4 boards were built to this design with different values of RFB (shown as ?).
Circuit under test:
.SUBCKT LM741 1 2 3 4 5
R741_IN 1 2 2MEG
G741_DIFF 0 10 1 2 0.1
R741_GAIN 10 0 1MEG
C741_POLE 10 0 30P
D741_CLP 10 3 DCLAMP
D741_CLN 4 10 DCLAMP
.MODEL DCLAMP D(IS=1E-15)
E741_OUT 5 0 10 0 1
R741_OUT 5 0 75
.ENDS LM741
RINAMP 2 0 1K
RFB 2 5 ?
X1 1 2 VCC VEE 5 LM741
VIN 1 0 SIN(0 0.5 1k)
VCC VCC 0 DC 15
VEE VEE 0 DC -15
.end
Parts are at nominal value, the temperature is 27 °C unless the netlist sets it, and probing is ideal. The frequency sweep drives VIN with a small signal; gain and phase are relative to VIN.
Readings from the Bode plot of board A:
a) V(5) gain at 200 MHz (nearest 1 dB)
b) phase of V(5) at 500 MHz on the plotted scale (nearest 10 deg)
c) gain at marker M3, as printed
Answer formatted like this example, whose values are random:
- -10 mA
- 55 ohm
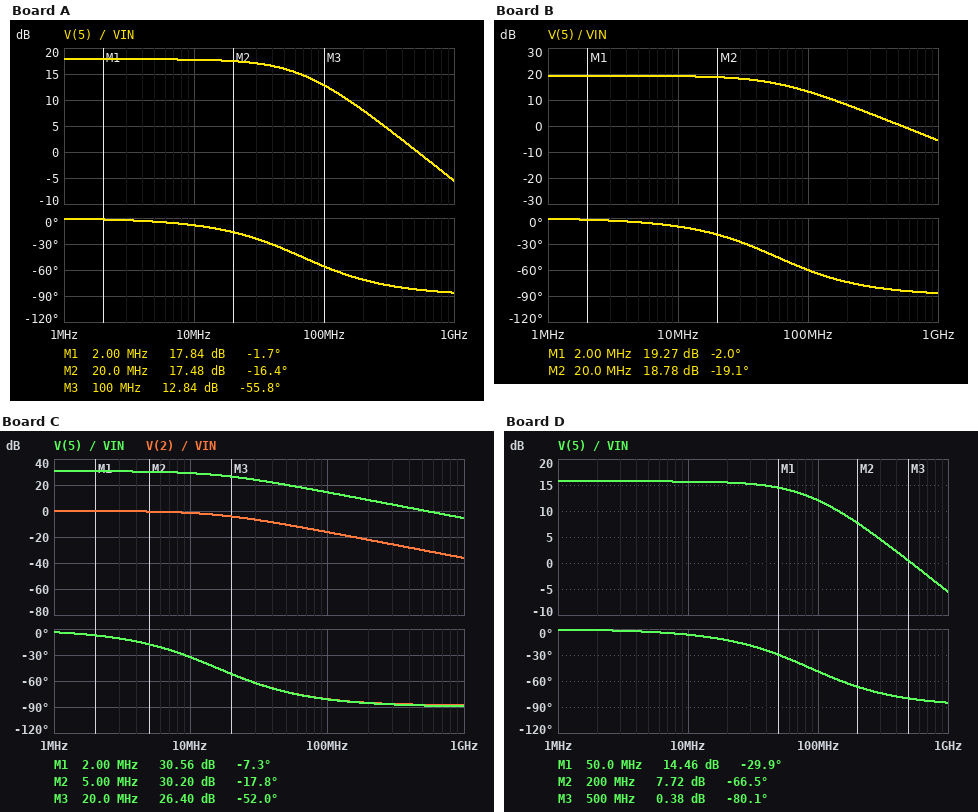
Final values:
- 8 dB
- -80 deg
- 12.84 dB
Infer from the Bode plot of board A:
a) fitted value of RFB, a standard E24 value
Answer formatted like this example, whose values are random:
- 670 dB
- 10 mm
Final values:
- 6.8 kΩ
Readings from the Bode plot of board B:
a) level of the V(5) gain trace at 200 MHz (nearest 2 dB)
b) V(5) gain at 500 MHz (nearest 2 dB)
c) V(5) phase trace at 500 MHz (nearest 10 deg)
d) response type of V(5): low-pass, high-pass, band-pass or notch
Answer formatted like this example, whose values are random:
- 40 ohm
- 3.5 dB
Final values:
- 8 dB
- 0 dB
- -80 deg
- low-pass
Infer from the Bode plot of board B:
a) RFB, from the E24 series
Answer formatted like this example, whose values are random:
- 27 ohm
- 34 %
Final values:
- 8.2 kΩ
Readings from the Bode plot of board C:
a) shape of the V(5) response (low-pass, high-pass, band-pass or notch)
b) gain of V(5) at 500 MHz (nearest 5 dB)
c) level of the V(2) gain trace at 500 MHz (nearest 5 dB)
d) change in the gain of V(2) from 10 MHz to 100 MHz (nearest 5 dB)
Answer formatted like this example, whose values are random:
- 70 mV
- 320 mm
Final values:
- low-pass
- 0 dB
- -30 dB
- -15 dB
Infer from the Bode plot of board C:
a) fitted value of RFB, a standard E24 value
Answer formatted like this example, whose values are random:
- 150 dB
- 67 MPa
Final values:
- 33 kΩ
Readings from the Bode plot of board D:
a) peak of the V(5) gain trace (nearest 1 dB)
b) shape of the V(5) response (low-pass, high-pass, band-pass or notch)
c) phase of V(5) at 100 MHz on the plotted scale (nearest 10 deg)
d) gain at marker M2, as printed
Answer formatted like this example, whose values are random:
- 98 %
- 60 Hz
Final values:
- 16 dB
- low-pass
- -50 deg
- 7.72 dB
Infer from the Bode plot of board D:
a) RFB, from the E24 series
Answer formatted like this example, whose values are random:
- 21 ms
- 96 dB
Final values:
- 5.1 kΩ
